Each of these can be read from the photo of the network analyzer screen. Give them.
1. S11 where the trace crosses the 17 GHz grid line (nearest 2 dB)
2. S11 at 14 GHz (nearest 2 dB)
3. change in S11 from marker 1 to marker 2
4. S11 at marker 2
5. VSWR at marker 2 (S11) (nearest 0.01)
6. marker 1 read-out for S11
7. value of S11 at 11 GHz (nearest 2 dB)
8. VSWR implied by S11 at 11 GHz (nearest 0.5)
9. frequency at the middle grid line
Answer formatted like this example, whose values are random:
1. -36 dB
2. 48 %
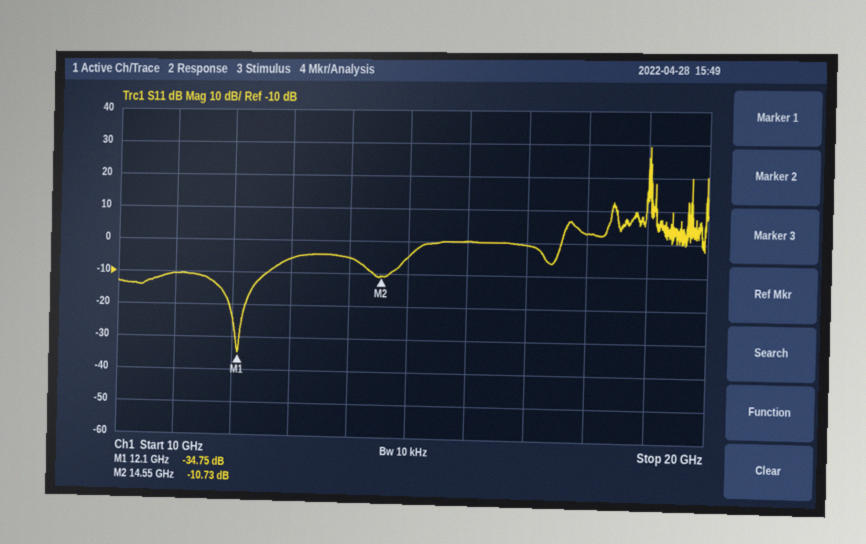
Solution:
1. 0 dB
2. -6 dB
3. 24.02 dB
4. -10.73 dB
5. 1.82
6. -34.75 dB
7. -10 dB
8. 2.0
9. 15 GHz
